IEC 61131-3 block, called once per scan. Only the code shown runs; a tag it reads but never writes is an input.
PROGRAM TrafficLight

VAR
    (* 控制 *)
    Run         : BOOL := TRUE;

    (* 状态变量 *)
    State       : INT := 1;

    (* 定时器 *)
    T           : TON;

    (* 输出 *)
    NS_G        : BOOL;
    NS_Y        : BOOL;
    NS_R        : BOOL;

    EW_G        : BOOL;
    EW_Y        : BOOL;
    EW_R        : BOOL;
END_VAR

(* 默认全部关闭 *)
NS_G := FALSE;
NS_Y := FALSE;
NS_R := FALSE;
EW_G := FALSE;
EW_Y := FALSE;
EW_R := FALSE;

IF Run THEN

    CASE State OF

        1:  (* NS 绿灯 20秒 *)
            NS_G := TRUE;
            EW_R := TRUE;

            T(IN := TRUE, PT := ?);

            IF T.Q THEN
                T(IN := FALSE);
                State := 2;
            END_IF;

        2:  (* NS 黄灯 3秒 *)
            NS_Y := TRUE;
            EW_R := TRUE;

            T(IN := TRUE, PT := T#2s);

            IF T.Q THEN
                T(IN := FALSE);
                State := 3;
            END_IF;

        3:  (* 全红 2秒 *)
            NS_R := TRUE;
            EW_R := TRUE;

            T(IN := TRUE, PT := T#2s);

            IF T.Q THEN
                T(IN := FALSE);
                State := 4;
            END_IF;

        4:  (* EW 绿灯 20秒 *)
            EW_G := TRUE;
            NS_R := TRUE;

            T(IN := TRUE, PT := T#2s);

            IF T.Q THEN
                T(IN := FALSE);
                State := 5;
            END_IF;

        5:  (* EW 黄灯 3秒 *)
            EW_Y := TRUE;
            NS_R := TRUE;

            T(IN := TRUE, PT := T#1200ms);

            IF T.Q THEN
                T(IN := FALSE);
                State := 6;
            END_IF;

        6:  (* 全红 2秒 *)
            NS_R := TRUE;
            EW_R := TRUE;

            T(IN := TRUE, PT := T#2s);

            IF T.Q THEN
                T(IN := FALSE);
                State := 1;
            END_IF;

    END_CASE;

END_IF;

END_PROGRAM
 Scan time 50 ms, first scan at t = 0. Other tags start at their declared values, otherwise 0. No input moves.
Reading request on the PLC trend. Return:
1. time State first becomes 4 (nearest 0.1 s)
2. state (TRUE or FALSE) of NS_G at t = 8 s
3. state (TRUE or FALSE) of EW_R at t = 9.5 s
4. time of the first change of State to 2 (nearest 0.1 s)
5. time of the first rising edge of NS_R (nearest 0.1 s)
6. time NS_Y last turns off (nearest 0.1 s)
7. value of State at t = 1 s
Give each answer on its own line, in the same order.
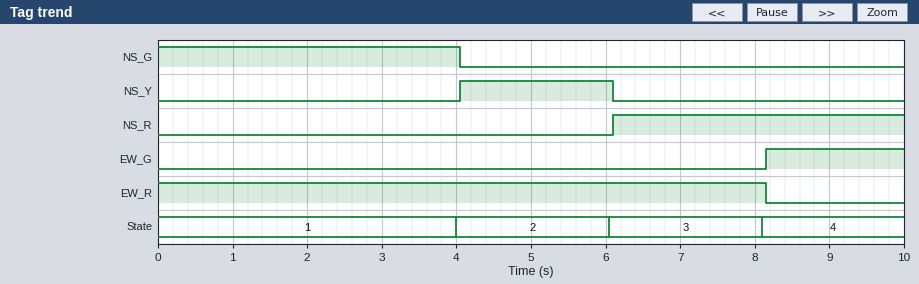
8.1 s
FALSE
FALSE
4.0 s
6.1 s
6.1 s
1
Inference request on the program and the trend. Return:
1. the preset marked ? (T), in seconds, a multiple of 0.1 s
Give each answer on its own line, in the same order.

4.0 s
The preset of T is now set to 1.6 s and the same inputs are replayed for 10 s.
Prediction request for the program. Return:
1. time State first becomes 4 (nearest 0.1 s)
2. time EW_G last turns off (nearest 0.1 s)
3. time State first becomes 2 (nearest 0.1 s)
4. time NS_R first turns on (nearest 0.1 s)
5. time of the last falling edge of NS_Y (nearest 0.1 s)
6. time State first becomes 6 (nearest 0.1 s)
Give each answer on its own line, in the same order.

5.7 s
7.8 s
1.6 s
3.7 s
3.7 s
9.0 s
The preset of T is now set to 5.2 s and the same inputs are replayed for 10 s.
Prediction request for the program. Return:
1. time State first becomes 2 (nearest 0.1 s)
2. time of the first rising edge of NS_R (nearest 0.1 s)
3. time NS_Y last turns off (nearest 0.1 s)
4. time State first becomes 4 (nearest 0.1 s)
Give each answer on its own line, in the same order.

5.2 s
7.3 s
7.3 s
9.3 s
